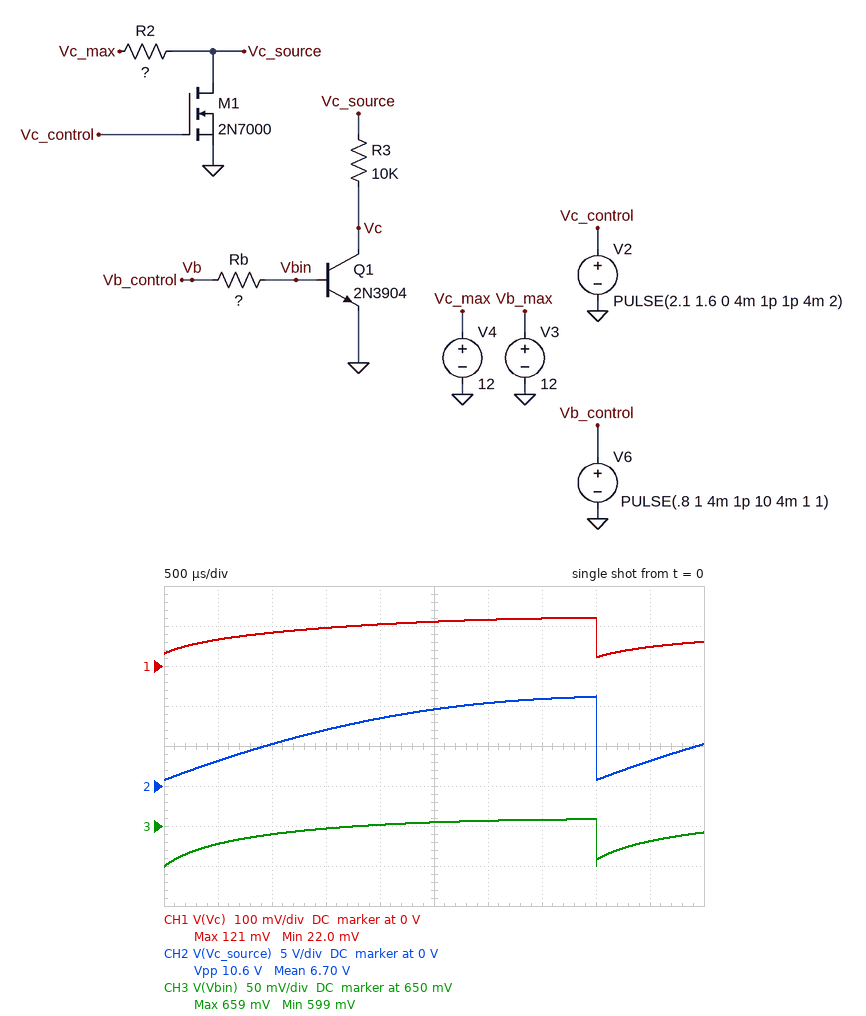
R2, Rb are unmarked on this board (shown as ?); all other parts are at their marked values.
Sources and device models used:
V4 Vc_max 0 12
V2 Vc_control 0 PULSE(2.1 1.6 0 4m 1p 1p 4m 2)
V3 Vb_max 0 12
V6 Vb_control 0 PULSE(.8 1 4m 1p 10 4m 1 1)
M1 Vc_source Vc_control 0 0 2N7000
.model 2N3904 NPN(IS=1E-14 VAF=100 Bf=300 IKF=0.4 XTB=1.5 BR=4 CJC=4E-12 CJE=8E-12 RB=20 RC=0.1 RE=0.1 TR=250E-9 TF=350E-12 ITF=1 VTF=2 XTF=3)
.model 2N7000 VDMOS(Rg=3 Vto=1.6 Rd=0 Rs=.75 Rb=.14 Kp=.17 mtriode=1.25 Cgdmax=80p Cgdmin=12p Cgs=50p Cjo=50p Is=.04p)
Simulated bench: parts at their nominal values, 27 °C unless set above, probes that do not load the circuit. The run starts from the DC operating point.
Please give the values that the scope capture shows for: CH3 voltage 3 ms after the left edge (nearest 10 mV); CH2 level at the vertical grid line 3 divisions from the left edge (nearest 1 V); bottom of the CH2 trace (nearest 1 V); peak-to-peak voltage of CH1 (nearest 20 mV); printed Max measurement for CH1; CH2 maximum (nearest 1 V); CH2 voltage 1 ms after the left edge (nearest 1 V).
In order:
660 mV
7 V
1 V
100 mV
121 mV
11 V
5 V
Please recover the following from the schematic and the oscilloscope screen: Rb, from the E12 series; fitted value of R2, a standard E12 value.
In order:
22 kΩ
560 Ω
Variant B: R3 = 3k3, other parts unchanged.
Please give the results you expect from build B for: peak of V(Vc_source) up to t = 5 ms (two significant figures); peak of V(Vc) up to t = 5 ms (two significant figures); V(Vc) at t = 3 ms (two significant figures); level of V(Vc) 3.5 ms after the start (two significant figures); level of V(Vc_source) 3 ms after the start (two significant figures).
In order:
11 V
4.7 V
3.9 V
4.4 V
9.9 V
